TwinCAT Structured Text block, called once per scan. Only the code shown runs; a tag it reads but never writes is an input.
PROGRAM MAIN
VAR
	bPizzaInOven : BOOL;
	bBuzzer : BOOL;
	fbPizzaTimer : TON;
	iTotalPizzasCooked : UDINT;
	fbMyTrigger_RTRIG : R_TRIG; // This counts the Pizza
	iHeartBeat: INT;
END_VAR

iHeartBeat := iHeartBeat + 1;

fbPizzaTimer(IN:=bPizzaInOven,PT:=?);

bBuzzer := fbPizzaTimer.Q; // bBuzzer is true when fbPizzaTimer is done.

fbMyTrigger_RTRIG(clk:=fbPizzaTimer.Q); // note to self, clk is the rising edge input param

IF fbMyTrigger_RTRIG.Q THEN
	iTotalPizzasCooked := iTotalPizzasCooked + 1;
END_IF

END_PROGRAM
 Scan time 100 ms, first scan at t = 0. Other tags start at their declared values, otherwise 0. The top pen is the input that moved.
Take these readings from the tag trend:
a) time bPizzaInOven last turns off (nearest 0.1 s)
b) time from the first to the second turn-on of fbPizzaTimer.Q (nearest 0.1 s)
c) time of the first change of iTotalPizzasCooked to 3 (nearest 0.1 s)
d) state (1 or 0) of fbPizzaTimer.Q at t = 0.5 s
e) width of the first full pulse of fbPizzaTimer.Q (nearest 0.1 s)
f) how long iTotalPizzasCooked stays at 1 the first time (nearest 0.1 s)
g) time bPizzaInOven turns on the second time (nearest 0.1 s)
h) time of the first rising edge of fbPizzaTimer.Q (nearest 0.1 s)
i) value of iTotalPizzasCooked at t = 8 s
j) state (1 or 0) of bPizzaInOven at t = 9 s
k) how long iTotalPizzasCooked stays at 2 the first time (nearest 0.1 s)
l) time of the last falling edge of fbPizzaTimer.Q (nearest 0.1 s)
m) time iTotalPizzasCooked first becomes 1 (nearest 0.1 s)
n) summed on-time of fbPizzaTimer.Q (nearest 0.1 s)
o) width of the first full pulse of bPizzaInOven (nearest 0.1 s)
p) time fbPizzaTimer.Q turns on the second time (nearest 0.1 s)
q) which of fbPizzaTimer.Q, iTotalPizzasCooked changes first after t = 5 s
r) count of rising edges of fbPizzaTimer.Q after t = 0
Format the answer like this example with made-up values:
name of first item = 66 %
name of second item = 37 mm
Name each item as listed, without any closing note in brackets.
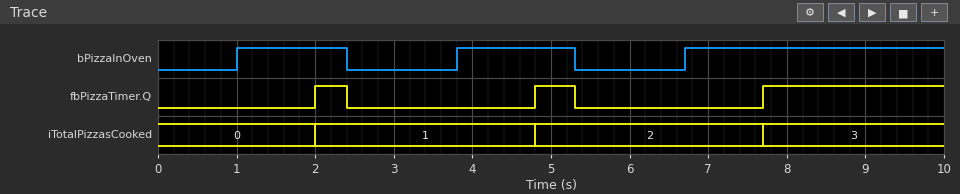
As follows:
time bPizzaInOven last turns off = 5.3 s
time from the first to the second turn-on of fbPizzaTimer.Q = 2.8 s
time of the first change of iTotalPizzasCooked to 3 = 7.7 s
state (1 or 0) of fbPizzaTimer.Q at t = 0.5 s = 0
width of the first full pulse of fbPizzaTimer.Q = 0.4 s
how long iTotalPizzasCooked stays at 1 the first time = 2.8 s
time bPizzaInOven turns on the second time = 3.8 s
time of the first rising edge of fbPizzaTimer.Q = 2.0 s
value of iTotalPizzasCooked at t = 8 s = 3
state (1 or 0) of bPizzaInOven at t = 9 s = 1
how long iTotalPizzasCooked stays at 2 the first time = 2.9 s
time of the last falling edge of fbPizzaTimer.Q = 5.3 s
time iTotalPizzasCooked first becomes 1 = 2.0 s
summed on-time of fbPizzaTimer.Q = 3.2 s
width of the first full pulse of bPizzaInOven = 1.4 s
time fbPizzaTimer.Q turns on the second time = 4.8 s
which of fbPizzaTimer.Q, iTotalPizzasCooked changes first after t = 5 s = fbPizzaTimer.Q
count of rising edges of fbPizzaTimer.Q after t = 0 = 3
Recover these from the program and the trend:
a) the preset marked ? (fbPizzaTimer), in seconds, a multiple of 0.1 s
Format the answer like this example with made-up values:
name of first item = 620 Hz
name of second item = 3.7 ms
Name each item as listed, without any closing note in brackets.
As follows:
the preset marked ? (fbPizzaTimer), in seconds, a multiple of 0.1 s = 1.0 s
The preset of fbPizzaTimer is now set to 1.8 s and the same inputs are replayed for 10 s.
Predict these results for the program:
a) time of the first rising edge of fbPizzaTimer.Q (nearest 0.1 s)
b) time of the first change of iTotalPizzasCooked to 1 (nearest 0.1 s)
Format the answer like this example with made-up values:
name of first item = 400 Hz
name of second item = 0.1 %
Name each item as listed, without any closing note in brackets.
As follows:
time of the first rising edge of fbPizzaTimer.Q = 8.5 s
time of the first change of iTotalPizzasCooked to 1 = 8.5 s
